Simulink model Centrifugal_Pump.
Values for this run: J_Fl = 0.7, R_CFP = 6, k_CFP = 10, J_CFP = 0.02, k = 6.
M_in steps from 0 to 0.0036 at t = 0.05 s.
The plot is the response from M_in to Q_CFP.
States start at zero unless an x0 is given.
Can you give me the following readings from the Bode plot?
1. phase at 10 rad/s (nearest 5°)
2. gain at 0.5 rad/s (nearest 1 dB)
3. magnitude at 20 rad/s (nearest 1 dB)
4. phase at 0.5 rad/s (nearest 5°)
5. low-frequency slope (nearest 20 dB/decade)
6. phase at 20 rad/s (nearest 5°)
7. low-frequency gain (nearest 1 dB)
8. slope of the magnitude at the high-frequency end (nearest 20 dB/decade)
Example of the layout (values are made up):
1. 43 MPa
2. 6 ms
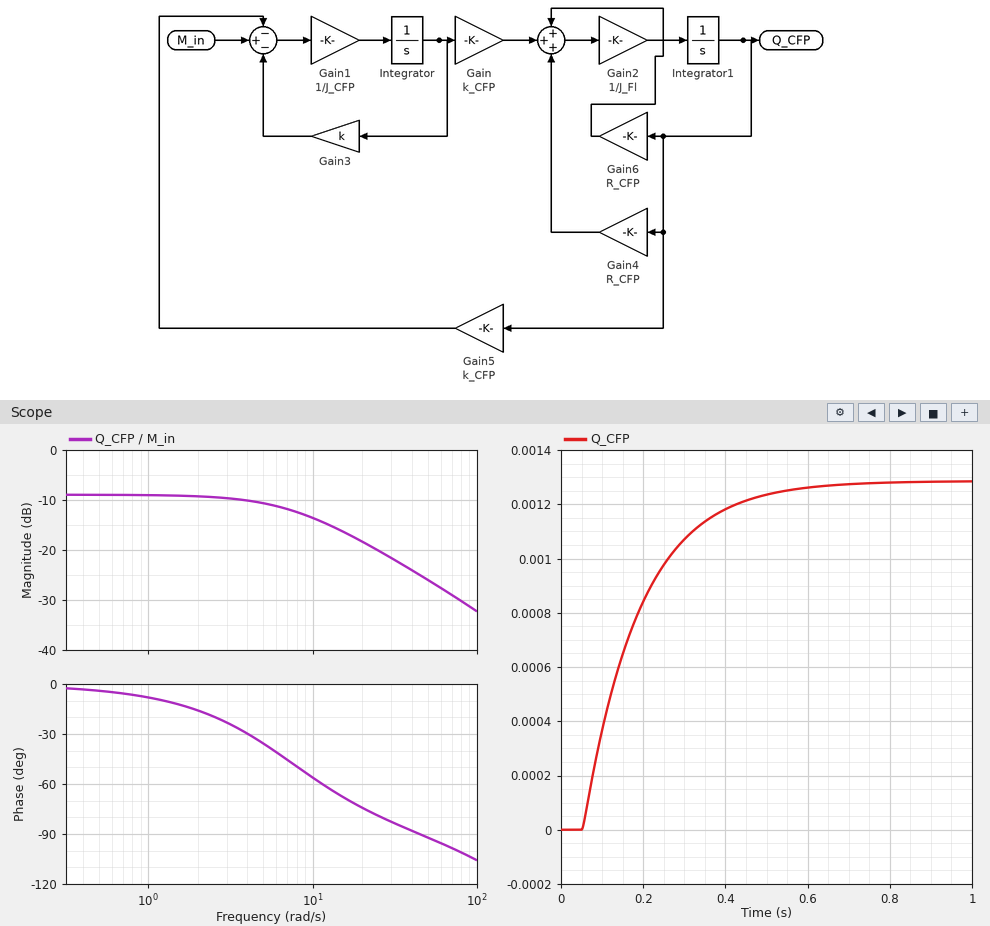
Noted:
1. -55°
2. -9 dB
3. -18 dB
4. -5°
5. 0 dB/decade
6. -75°
7. -9 dB
8. -20 dB/decade
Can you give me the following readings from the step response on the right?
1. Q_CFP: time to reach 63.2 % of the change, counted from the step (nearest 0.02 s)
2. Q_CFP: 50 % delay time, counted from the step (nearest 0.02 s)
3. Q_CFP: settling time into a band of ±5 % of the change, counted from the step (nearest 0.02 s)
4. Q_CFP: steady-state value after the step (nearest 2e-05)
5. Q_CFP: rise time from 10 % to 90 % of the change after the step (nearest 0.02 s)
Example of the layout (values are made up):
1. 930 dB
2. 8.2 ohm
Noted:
1. 0.14 s
2. 0.10 s
3. 0.42 s
4. 0.00128
5. 0.30 s
